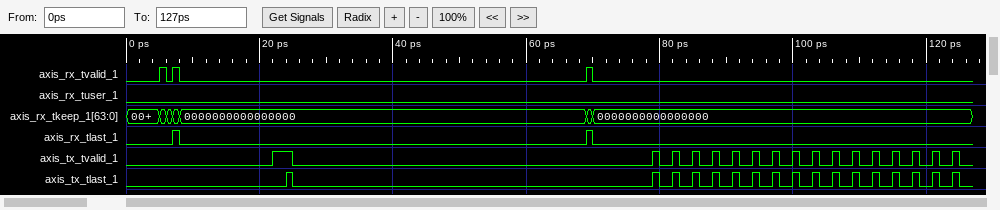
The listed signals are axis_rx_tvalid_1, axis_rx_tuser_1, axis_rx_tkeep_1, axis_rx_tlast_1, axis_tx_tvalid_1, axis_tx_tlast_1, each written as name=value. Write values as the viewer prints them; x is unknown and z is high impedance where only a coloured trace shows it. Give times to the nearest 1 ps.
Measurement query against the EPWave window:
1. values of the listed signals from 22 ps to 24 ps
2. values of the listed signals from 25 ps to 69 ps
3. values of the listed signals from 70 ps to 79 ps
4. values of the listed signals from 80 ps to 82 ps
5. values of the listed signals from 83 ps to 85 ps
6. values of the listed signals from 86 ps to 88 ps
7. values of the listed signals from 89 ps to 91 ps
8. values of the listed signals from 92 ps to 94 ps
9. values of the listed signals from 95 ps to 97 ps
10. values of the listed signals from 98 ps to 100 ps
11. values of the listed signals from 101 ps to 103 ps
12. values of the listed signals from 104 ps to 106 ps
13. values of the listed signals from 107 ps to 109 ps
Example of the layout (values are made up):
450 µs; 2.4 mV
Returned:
axis_rx_tvalid_1=0, axis_rx_tuser_1=0, axis_rx_tkeep_1=0000000000000000, axis_rx_tlast_1=0, axis_tx_tvalid_1=1, axis_tx_tlast_1=0; axis_rx_tvalid_1=0, axis_rx_tuser_1=0, axis_rx_tkeep_1=0000000000000000, axis_rx_tlast_1=0, axis_tx_tvalid_1=0, axis_tx_tlast_1=0; axis_rx_tvalid_1=0, axis_rx_tuser_1=0, axis_rx_tkeep_1=0000000000000000, axis_rx_tlast_1=0, axis_tx_tvalid_1=0, axis_tx_tlast_1=0; axis_rx_tvalid_1=0, axis_rx_tuser_1=0, axis_rx_tkeep_1=0000000000000000, axis_rx_tlast_1=0, axis_tx_tvalid_1=0, axis_tx_tlast_1=0; axis_rx_tvalid_1=0, axis_rx_tuser_1=0, axis_rx_tkeep_1=0000000000000000, axis_rx_tlast_1=0, axis_tx_tvalid_1=0, axis_tx_tlast_1=0; axis_rx_tvalid_1=0, axis_rx_tuser_1=0, axis_rx_tkeep_1=0000000000000000, axis_rx_tlast_1=0, axis_tx_tvalid_1=0, axis_tx_tlast_1=0; axis_rx_tvalid_1=0, axis_rx_tuser_1=0, axis_rx_tkeep_1=0000000000000000, axis_rx_tlast_1=0, axis_tx_tvalid_1=0, axis_tx_tlast_1=0; axis_rx_tvalid_1=0, axis_rx_tuser_1=0, axis_rx_tkeep_1=0000000000000000, axis_rx_tlast_1=0, axis_tx_tvalid_1=0, axis_tx_tlast_1=0; axis_rx_tvalid_1=0, axis_rx_tuser_1=0, axis_rx_tkeep_1=0000000000000000, axis_rx_tlast_1=0, axis_tx_tvalid_1=0, axis_tx_tlast_1=0; axis_rx_tvalid_1=0, axis_rx_tuser_1=0, axis_rx_tkeep_1=0000000000000000, axis_rx_tlast_1=0, axis_tx_tvalid_1=0, axis_tx_tlast_1=0; axis_rx_tvalid_1=0, axis_rx_tuser_1=0, axis_rx_tkeep_1=0000000000000000, axis_rx_tlast_1=0, axis_tx_tvalid_1=0, axis_tx_tlast_1=0; axis_rx_tvalid_1=0, axis_rx_tuser_1=0, axis_rx_tkeep_1=0000000000000000, axis_rx_tlast_1=0, axis_tx_tvalid_1=0, axis_tx_tlast_1=0; axis_rx_tvalid_1=0, axis_rx_tuser_1=0, axis_rx_tkeep_1=0000000000000000, axis_rx_tlast_1=0, axis_tx_tvalid_1=0, axis_tx_tlast_1=0
